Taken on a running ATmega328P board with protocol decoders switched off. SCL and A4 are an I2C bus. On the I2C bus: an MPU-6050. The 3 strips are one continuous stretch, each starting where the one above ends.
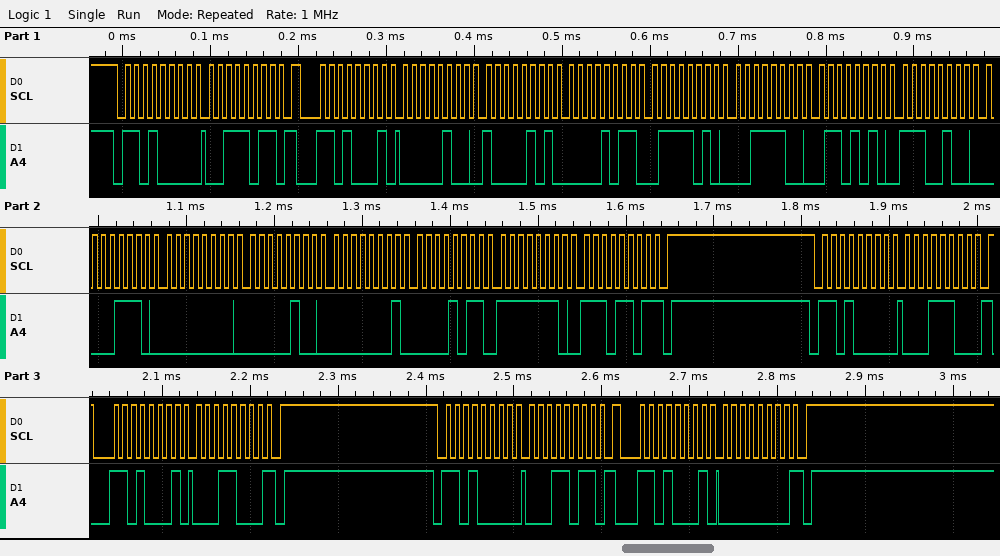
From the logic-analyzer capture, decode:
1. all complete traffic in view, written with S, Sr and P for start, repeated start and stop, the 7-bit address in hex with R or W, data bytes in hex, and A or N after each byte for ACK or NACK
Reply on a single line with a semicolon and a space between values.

S 68W A 3B A Sr 68R A 04 A 85 A 0B A 7A A 3C A 6A A E4 A 0E A 00 A 04 A 01 A 0B A FE A ED N P S 68W A 1C A Sr 68R A 18 N P S 68W A 1B A Sr 68R A 00 N P
